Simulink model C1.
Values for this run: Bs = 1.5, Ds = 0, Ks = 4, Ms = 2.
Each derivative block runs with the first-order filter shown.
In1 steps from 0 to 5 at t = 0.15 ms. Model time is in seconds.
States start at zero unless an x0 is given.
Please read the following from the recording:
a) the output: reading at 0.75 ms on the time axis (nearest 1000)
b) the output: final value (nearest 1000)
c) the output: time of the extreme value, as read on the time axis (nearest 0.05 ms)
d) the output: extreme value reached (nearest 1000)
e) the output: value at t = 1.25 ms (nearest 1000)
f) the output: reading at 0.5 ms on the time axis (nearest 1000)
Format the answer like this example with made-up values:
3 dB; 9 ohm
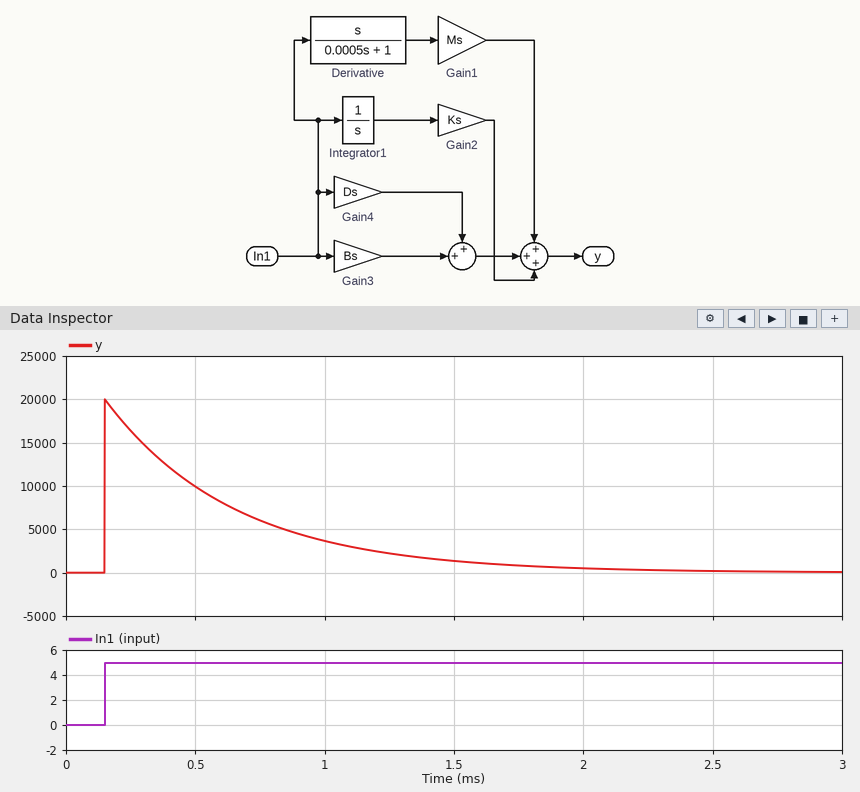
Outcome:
6000; 0; 0.15 ms; 20000; 2000; 10000
